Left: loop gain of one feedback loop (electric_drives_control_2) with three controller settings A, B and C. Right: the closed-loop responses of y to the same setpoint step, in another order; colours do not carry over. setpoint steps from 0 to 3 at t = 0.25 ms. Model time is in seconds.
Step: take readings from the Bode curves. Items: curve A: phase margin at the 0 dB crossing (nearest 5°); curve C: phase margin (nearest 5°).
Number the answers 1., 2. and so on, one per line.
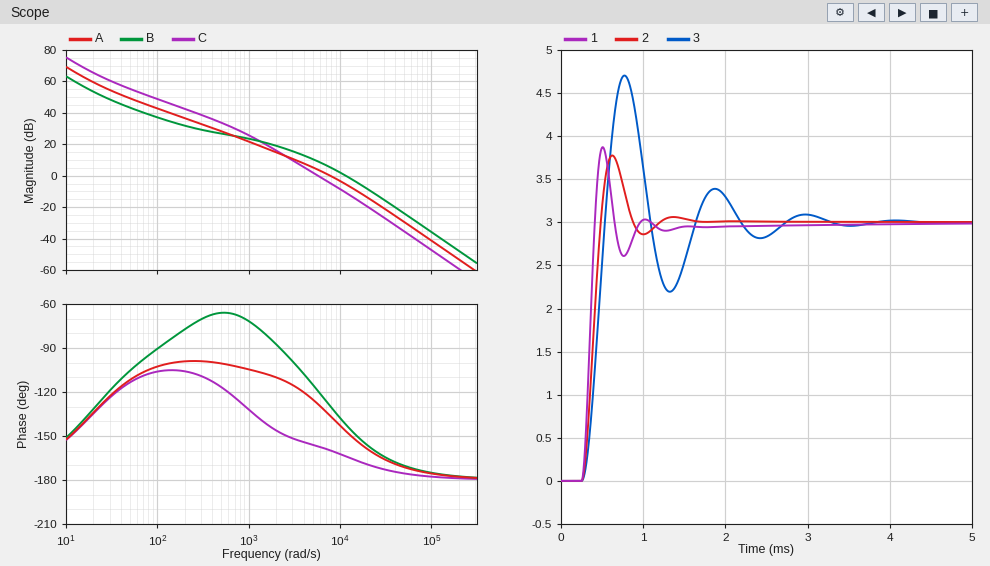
1. 45°
2. 25°
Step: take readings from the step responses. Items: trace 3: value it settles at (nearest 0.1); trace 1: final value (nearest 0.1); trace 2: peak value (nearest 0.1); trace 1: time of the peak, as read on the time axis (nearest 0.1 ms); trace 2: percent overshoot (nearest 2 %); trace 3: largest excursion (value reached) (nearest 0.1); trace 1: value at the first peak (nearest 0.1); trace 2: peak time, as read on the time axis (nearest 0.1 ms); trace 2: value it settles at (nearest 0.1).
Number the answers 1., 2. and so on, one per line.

1. 3.0
2. 3.0
3. 3.8
4. 0.5 ms
5. 26 %
6. 4.7
7. 3.9
8. 0.6 ms
9. 3.0
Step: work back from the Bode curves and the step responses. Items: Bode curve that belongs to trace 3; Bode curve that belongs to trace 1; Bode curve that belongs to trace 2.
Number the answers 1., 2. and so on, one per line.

1. C
2. B
3. A
